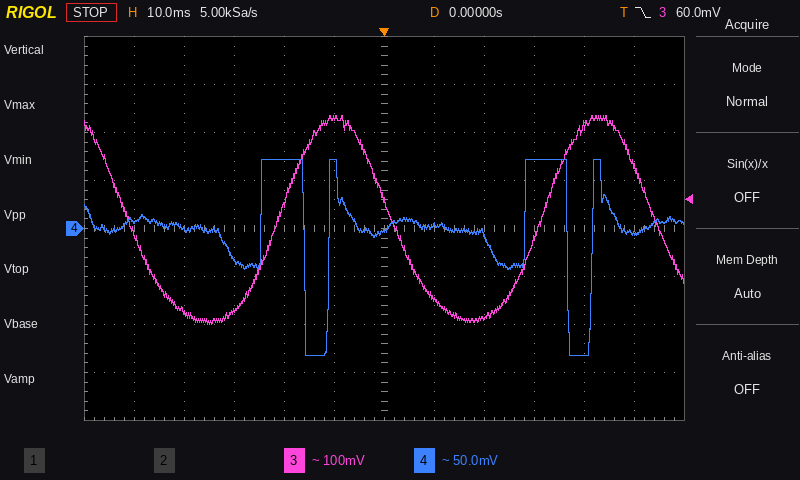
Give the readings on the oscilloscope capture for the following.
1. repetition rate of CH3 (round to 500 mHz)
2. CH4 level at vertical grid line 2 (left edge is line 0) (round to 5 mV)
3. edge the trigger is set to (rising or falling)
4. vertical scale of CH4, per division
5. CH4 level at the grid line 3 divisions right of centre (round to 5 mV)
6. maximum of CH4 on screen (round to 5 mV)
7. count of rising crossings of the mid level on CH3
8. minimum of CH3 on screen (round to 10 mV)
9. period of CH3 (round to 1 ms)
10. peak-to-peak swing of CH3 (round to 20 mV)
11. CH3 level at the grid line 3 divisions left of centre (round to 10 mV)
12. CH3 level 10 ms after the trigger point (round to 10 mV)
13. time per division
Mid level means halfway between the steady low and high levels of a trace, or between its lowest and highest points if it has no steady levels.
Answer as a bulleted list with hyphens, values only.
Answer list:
- 19.0 Hz
- 0 mV
- falling
- 50 mV
- 70 mV
- 70 mV
- 2
- -200 mV
- 53 ms
- 440 mV
- -170 mV
- -150 mV
- 10 ms
